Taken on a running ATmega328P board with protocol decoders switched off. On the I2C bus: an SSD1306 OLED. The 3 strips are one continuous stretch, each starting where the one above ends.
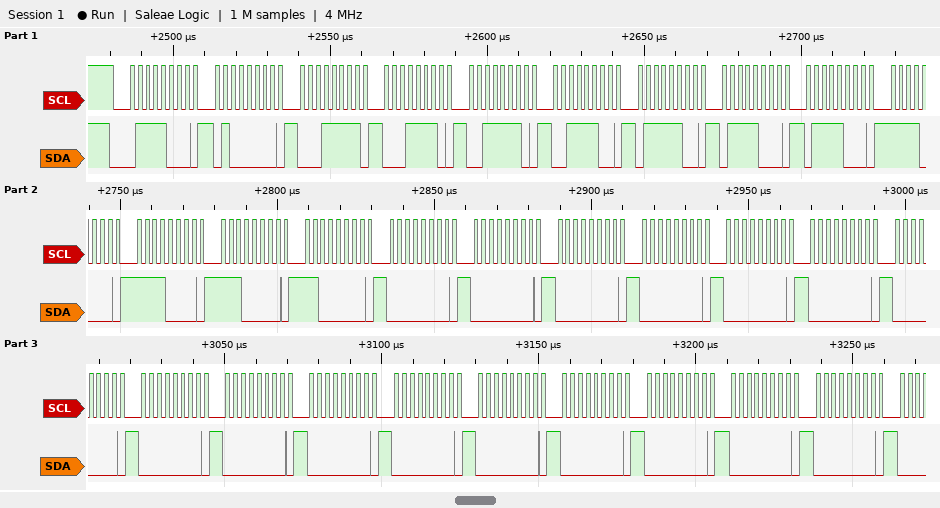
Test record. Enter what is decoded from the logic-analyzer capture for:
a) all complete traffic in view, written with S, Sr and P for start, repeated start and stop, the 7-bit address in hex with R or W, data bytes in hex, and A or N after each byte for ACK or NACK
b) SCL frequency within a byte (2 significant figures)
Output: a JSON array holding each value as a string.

["S 3CW A 40 A 1F A 1E A 3E A 3C A 7C A 78 A 78 A F0 A F0 A E0 A C0 A 00 A 00 A 00 A 00 A 00 A 00 A 00 A 00 A 00 A 00 A 00 A 00 A 00 A 00 A 00 A 00 A", "400 kHz"]
